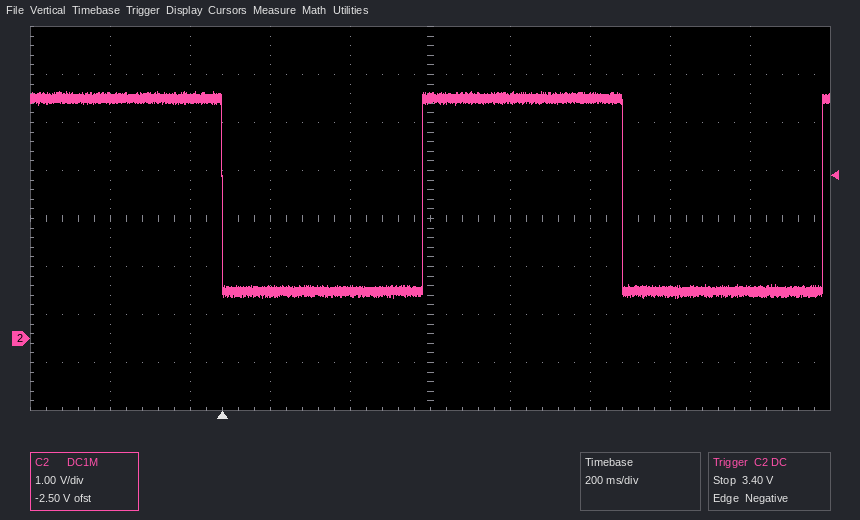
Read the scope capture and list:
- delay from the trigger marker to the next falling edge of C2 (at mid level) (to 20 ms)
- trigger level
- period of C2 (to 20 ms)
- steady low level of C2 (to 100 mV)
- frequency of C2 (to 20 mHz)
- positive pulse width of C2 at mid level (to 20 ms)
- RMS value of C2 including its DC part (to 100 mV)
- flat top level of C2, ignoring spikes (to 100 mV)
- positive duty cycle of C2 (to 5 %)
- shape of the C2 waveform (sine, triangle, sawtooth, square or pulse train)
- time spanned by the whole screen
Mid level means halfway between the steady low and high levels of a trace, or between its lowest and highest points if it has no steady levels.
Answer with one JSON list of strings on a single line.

["1.00 s", "3.40 V", "1.00 s", "1.0 V", "1.00 Hz", "500 ms", "3.6 V", "5.0 V", "50 %", "square", "2 s"]
